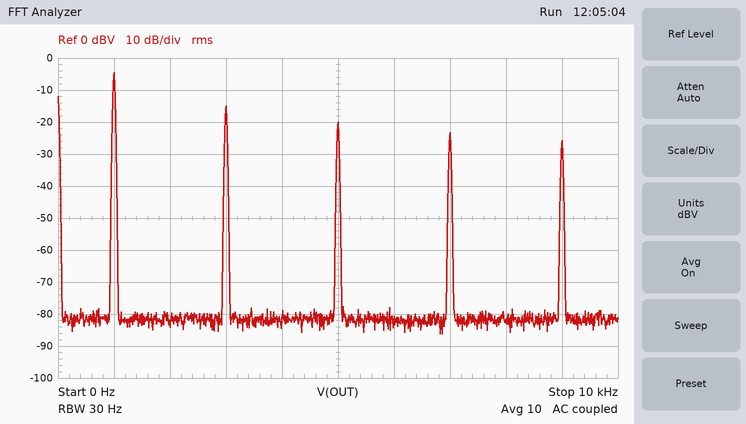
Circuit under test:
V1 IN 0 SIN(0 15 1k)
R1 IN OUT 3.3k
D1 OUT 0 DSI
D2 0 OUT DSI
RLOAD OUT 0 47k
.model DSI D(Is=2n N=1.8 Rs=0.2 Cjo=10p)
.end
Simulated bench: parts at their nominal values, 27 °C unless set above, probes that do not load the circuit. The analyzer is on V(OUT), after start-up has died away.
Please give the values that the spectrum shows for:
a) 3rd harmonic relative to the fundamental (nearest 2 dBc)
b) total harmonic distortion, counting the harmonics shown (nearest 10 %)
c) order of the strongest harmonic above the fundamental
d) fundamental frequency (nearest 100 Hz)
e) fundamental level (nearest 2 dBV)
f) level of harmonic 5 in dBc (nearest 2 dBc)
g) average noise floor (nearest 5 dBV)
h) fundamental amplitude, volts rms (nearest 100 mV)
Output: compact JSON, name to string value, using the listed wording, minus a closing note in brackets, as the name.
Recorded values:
{"3rd harmonic relative to the fundamental": "-10 dBc", "total harmonic distortion, counting the harmonics shown": "40 %", "order of the strongest harmonic above the fundamental": "3", "fundamental frequency": "1.0 kHz", "fundamental level": "-4 dBV", "level of harmonic 5 in dBc": "-16 dBc", "average noise floor": "-80 dBV", "fundamental amplitude, volts rms": "600 mV"}
